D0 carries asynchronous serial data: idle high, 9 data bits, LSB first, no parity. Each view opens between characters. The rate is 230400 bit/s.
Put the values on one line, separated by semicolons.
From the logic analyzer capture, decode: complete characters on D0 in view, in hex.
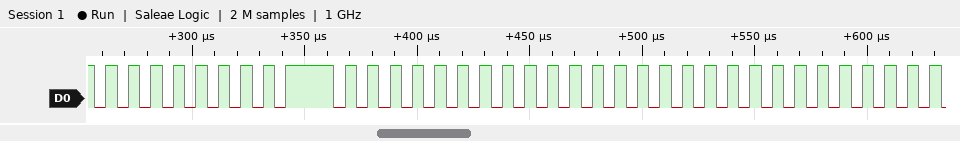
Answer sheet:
AD, 1AD, AD, AD, AD, AD, AD
